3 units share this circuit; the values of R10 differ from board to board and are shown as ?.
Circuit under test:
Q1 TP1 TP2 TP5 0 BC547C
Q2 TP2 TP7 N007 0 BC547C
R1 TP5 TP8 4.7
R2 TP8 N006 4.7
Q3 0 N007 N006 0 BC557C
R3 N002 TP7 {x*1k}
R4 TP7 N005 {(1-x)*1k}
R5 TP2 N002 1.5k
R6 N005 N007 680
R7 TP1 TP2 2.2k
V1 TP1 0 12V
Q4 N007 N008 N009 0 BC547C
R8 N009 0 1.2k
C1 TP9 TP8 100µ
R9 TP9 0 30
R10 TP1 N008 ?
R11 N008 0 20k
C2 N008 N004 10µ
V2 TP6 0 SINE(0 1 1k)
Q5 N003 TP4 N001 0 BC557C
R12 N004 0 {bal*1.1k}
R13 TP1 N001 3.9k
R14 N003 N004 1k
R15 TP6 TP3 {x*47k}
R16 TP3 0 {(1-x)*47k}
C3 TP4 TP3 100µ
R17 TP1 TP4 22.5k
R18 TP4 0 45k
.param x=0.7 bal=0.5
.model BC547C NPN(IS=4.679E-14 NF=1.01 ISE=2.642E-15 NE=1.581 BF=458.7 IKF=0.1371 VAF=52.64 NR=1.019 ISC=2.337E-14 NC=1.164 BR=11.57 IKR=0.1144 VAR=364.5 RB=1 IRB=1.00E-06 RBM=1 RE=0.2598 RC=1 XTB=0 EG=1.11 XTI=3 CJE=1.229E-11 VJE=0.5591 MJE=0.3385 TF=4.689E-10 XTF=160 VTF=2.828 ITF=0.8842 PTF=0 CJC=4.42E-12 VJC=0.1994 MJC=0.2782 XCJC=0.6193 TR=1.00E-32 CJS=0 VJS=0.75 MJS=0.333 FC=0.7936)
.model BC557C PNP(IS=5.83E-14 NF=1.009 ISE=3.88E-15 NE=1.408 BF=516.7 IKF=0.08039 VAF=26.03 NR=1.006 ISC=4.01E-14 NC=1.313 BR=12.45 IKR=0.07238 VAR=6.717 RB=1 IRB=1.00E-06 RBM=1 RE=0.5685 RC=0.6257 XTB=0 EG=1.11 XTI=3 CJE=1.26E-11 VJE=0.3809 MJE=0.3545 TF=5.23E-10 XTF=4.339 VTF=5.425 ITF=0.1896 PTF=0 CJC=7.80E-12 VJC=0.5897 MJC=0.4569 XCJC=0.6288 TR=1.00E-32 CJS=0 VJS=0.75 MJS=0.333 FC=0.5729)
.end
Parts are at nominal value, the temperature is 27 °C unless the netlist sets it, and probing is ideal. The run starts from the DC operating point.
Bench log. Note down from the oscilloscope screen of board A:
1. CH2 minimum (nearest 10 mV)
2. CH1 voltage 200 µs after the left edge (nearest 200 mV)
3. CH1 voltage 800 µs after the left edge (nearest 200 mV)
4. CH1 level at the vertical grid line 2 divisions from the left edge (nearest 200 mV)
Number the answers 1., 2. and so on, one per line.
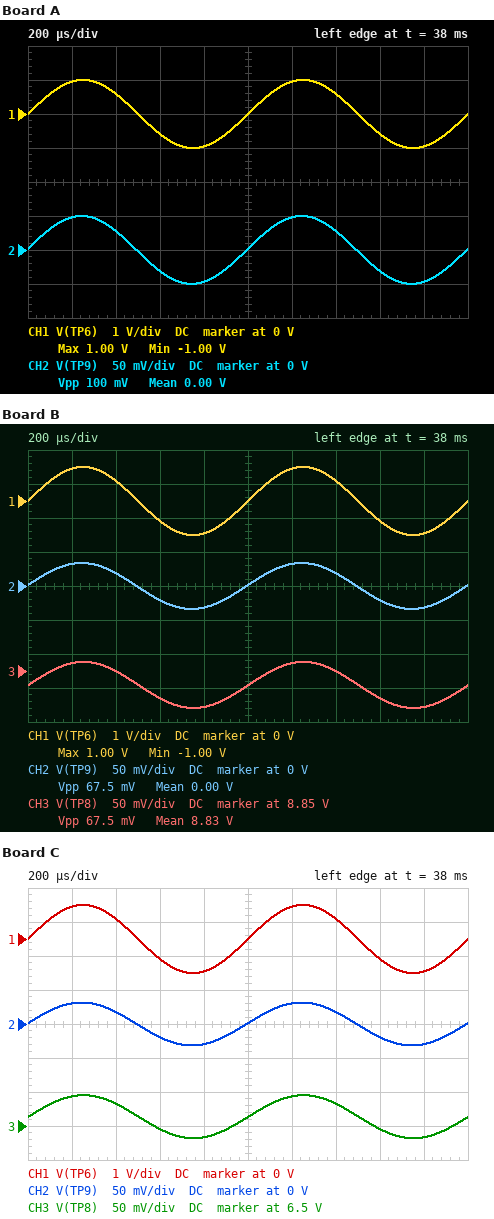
1. -50 mV
2. 1.0 V
3. -1.0 V
4. 600 mV
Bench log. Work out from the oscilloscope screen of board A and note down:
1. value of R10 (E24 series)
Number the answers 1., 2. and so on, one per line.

1. 180 kΩ
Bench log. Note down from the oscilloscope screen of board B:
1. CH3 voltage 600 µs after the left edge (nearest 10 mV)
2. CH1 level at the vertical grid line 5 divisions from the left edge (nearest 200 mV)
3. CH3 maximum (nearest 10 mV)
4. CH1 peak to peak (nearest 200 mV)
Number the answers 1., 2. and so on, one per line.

1. 8.81 V
2. 0 V
3. 8.86 V
4. 2.0 V
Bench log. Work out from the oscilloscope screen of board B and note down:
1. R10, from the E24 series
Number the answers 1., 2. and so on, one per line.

1. 110 kΩ
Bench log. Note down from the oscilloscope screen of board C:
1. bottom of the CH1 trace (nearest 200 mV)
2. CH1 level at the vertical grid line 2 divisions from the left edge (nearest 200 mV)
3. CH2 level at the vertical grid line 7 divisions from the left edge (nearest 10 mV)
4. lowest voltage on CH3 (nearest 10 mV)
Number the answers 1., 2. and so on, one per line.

1. -1.0 V
2. 600 mV
3. 20 mV
4. 6.48 V
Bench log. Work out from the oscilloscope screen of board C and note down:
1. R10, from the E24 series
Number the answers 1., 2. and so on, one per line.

1. 56 kΩ
